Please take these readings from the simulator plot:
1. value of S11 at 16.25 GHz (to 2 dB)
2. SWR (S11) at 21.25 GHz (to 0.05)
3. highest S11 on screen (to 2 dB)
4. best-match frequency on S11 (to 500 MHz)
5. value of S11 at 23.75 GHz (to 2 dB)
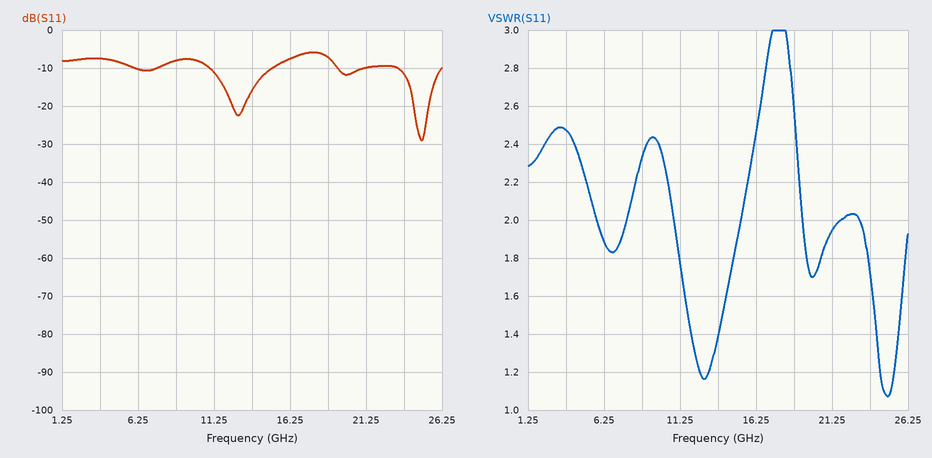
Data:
-8 dB
1.95
-6 dB
25.0 GHz
-12 dB
